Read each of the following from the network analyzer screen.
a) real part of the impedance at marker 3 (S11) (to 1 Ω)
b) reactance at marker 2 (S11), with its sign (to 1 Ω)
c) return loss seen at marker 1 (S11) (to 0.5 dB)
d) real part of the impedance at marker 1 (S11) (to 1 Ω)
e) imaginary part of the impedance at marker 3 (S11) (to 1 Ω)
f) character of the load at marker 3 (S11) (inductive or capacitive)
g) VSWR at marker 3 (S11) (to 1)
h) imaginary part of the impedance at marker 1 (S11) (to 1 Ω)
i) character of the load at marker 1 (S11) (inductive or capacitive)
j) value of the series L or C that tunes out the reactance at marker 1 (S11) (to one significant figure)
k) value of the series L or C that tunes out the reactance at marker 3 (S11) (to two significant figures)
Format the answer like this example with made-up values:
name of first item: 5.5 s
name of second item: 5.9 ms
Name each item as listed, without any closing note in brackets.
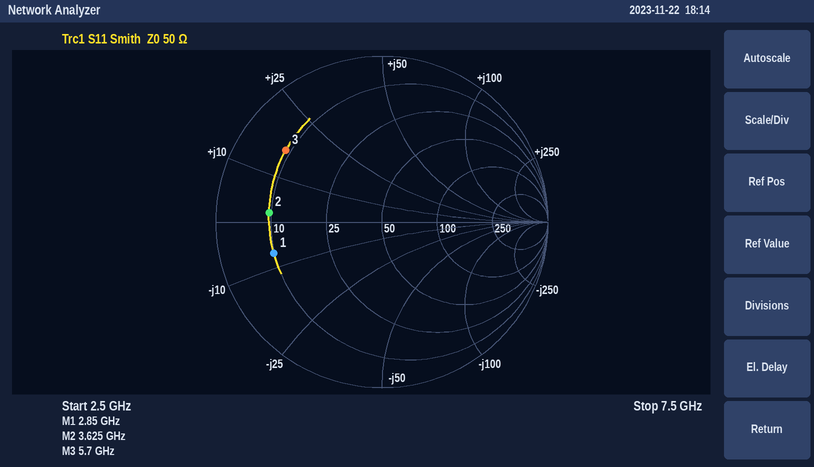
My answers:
real part of the impedance at marker 3 (S11): 9 Ω
reactance at marker 2 (S11), with its sign: +2 Ω
return loss seen at marker 1 (S11): 3.5 dB
real part of the impedance at marker 1 (S11): 10 Ω
imaginary part of the impedance at marker 3 (S11): +16 Ω
character of the load at marker 3 (S11): inductive
VSWR at marker 3 (S11): 6
imaginary part of the impedance at marker 1 (S11): -7 Ω
character of the load at marker 1 (S11): capacitive
value of the series L or C that tunes out the reactance at marker 1 (S11): 400 pH
value of the series L or C that tunes out the reactance at marker 3 (S11): 1.7 pF
